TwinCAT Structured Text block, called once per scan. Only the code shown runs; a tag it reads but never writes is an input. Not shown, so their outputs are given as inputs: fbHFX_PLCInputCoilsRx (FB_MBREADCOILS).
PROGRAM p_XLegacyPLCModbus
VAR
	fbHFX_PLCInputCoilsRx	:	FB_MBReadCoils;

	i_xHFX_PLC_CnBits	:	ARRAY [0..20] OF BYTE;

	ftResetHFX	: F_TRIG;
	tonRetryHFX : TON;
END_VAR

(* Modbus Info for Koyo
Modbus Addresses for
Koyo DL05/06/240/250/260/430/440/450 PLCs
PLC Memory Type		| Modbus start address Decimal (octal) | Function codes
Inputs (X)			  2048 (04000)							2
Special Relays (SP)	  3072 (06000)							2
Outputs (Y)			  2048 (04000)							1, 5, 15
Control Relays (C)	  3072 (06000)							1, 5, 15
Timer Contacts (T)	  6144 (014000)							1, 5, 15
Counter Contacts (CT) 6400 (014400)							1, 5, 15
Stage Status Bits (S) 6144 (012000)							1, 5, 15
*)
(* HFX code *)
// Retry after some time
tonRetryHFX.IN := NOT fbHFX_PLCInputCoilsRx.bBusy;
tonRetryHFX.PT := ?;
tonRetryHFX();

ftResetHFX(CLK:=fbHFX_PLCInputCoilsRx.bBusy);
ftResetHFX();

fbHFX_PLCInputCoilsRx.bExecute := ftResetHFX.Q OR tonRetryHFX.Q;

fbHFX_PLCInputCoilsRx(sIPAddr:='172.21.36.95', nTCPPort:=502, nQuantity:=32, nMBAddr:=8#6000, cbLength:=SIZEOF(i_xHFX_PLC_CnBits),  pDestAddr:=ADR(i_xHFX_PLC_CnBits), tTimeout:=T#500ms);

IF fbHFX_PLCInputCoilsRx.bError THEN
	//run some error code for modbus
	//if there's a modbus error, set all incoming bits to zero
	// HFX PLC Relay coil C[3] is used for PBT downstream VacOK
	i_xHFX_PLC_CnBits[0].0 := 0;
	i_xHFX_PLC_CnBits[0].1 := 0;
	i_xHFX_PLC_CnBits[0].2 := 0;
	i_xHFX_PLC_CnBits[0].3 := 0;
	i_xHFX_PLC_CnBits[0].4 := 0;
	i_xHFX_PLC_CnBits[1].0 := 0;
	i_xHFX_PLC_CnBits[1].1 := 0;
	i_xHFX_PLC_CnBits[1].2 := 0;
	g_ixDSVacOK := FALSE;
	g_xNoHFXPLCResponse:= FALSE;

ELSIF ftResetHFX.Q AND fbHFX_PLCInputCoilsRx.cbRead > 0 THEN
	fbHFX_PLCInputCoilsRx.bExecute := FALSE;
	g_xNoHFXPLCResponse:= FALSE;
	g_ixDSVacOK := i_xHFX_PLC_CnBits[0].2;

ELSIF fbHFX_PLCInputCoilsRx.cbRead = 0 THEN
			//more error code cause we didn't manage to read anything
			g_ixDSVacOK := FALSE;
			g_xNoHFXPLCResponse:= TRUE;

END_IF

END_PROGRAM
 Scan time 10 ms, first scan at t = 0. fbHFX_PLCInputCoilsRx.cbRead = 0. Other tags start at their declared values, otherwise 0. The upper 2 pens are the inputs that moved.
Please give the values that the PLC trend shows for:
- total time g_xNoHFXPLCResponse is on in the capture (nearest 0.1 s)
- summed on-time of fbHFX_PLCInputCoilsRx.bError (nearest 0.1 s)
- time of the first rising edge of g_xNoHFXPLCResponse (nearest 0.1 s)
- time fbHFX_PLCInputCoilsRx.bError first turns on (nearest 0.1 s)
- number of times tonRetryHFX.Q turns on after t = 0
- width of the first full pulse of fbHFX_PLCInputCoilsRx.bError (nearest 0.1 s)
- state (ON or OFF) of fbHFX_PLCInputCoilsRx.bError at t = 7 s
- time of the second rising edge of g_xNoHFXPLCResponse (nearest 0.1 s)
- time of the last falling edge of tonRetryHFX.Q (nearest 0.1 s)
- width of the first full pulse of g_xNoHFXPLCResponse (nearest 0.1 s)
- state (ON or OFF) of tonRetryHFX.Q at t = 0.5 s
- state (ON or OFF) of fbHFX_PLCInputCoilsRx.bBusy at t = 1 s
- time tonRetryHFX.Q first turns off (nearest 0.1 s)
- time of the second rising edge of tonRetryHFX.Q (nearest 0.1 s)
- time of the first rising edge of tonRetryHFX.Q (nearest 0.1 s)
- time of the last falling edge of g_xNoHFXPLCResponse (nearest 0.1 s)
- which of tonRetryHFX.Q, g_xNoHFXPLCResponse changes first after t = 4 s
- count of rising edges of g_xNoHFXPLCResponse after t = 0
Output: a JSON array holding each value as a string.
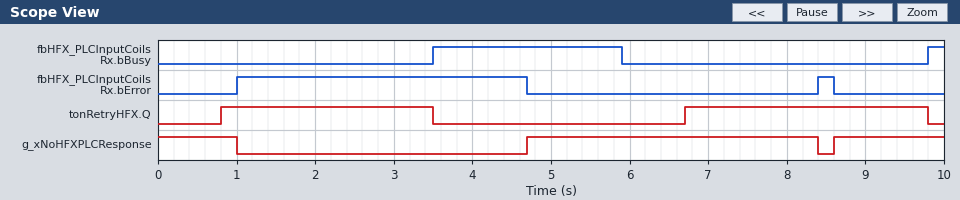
["6.1 s", "3.9 s", "4.7 s", "1.0 s", "2", "3.7 s", "OFF", "8.6 s", "9.8 s", "3.7 s", "OFF", "OFF", "3.5 s", "6.7 s", "0.8 s", "8.4 s", "g_xNoHFXPLCResponse", "2"]
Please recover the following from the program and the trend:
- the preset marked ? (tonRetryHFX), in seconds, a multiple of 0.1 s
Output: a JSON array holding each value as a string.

["0.8 s"]
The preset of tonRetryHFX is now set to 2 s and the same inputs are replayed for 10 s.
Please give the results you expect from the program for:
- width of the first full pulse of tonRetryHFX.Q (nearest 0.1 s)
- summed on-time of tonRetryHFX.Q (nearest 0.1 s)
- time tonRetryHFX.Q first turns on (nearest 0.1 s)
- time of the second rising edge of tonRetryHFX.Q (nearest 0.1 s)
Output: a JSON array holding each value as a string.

["1.5 s", "3.4 s", "2.0 s", "7.9 s"]
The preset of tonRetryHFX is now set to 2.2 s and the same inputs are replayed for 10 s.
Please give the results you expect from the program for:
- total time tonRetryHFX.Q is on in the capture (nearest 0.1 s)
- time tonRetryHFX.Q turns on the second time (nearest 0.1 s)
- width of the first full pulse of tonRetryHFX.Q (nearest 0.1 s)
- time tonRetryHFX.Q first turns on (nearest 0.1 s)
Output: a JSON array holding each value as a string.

["3.0 s", "8.1 s", "1.3 s", "2.2 s"]
